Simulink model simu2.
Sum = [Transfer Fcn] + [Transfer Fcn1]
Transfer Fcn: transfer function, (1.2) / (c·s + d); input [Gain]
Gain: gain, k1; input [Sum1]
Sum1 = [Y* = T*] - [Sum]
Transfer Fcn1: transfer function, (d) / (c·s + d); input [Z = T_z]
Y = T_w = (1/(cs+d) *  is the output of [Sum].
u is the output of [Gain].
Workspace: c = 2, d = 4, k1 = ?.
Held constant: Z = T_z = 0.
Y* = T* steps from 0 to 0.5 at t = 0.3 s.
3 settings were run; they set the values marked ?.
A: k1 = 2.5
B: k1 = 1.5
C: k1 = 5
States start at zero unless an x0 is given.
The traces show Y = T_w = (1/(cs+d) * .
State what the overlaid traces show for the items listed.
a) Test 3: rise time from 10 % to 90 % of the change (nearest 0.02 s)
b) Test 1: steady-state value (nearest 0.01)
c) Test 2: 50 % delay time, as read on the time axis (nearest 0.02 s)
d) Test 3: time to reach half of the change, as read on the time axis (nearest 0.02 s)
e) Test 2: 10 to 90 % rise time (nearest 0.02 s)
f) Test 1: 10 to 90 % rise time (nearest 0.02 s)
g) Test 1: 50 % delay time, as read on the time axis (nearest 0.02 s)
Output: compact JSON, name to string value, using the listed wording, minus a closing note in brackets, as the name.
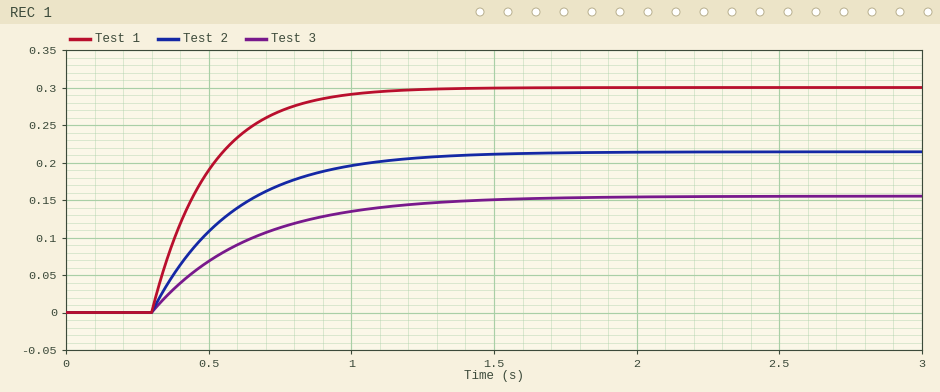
{"Test 3: rise time from 10 % to 90 % of the change": "0.76 s", "Test 1: steady-state value": "0.30", "Test 2: 50 % delay time, as read on the time axis": "0.50 s", "Test 3: time to reach half of the change, as read on the time axis": "0.54 s", "Test 2: 10 to 90 % rise time": "0.62 s", "Test 1: 10 to 90 % rise time": "0.44 s", "Test 1: 50 % delay time, as read on the time axis": "0.44 s"}
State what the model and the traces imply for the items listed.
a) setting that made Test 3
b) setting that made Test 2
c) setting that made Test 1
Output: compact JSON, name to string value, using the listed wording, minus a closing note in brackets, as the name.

{"setting that made Test 3": "B", "setting that made Test 2": "A", "setting that made Test 1": "C"}
